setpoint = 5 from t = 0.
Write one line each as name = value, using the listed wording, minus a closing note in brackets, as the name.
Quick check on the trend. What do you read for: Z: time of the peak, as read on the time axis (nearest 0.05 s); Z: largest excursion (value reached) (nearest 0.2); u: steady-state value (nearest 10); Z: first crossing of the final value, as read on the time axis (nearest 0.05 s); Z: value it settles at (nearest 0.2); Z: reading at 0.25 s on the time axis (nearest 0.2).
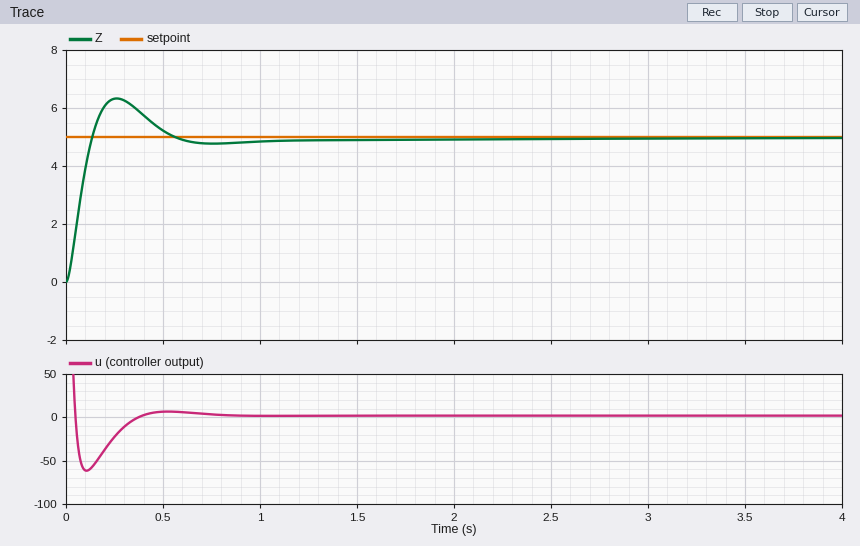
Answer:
Z: time of the peak, as read on the time axis = 0.25 s
Z: largest excursion (value reached) = 6.4
u: steady-state value = 0
Z: first crossing of the final value, as read on the time axis = 0.15 s
Z: value it settles at = 5.0
Z: reading at 0.25 s on the time axis = 6.4
